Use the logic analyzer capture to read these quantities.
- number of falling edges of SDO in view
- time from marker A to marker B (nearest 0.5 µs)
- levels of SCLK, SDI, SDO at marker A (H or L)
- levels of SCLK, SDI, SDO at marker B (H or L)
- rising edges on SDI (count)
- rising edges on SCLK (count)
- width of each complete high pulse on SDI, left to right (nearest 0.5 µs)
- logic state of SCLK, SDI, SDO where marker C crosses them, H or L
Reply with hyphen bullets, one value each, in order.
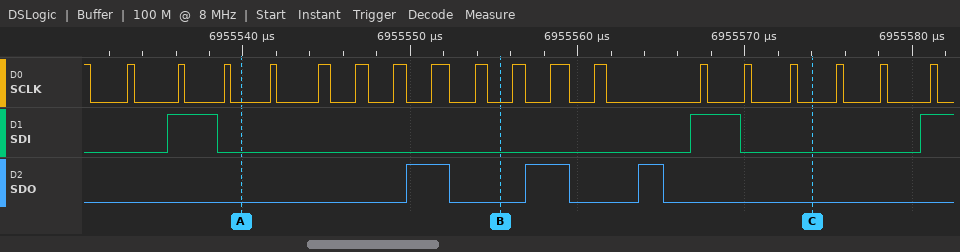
- 3
- 15.5 µs
- SCLK=L, SDI=L, SDO=L
- SCLK=L, SDI=L, SDO=L
- 3
- 18
- 3 µs, 3 µs
- SCLK=L, SDI=L, SDO=L
